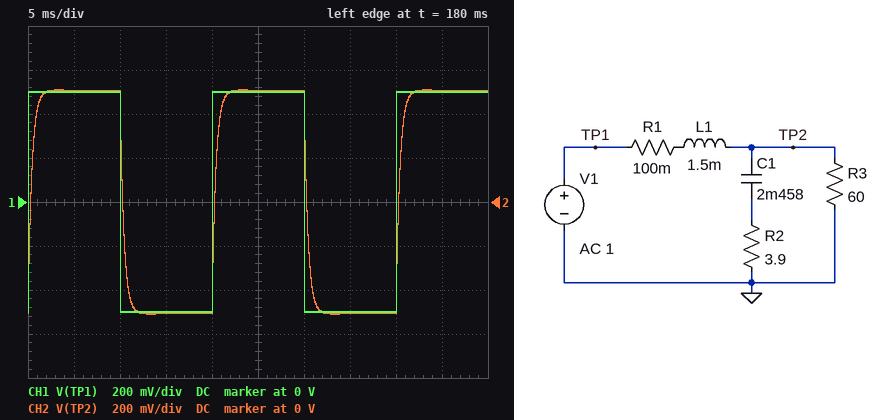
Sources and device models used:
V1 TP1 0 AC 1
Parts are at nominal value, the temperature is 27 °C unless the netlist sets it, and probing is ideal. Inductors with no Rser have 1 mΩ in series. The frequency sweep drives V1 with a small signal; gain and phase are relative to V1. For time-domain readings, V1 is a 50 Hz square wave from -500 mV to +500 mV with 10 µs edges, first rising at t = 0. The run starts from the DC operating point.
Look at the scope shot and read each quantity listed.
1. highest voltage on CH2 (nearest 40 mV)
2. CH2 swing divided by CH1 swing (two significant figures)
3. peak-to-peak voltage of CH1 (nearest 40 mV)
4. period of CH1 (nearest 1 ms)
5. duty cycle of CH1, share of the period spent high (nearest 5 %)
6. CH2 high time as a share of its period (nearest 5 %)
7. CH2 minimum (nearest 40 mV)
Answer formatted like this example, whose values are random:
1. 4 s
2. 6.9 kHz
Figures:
1. 520 mV
2. 1.0
3. 1.00 V
4. 20 ms
5. 50 %
6. 50 %
7. -520 mV
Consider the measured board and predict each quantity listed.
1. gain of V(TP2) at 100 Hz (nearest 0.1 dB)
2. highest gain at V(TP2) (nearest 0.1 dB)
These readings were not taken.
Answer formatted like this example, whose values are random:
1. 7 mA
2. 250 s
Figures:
1. -0.2 dB
2. 0.1 dB
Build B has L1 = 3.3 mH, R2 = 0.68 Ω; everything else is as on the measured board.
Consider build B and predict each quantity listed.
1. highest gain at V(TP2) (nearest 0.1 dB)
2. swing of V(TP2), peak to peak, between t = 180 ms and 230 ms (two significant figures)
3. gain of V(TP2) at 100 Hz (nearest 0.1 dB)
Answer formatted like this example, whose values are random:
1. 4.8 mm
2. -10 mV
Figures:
1. 4.8 dB
2. 2.1 V
3. -4.9 dB
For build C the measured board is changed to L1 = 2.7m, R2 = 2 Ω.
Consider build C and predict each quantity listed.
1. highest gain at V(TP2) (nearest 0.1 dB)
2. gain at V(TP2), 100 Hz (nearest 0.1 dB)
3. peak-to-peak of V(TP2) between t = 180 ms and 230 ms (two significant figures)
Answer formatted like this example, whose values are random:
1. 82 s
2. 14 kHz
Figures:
1. 0.9 dB
2. -1.1 dB
3. 1.2 V
